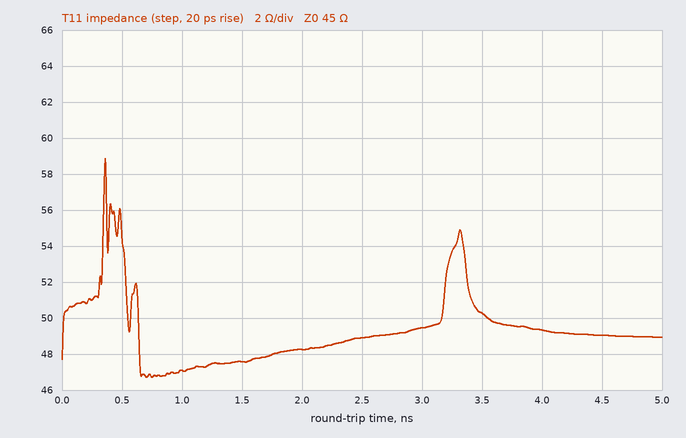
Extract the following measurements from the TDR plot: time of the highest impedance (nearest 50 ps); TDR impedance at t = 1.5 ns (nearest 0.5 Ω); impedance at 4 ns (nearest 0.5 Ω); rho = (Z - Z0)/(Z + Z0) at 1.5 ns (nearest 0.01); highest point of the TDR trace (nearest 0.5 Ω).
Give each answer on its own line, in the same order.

350 ps
47.5 Ω
49.5 Ω
+0.03
59.0 Ω
